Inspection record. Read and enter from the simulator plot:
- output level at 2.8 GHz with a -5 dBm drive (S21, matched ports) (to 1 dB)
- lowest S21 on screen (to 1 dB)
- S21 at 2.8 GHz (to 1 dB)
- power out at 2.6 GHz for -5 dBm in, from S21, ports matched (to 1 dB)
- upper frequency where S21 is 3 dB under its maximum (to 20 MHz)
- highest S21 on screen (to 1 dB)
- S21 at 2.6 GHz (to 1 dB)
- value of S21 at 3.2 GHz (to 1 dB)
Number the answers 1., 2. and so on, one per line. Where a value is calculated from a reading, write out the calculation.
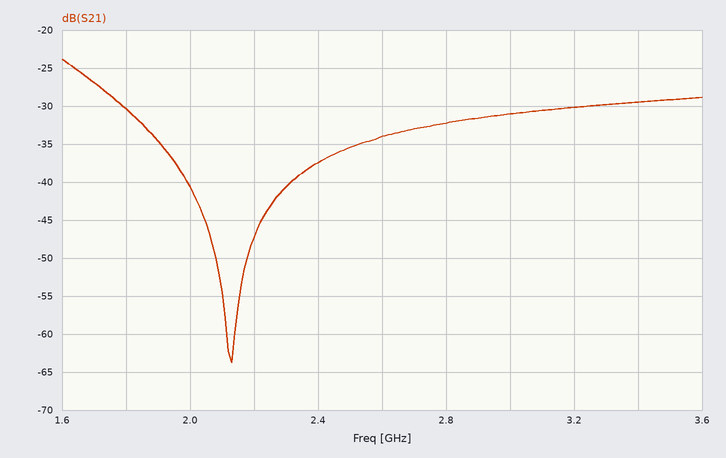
1. -5 dBm + (-32 dB) = -37 dBm
2. -64 dB
3. -32 dB
4. -5 dBm + (-34 dB) = -39 dBm
5. 1.70 GHz
6. -24 dB
7. -34 dB
8. -30 dB
